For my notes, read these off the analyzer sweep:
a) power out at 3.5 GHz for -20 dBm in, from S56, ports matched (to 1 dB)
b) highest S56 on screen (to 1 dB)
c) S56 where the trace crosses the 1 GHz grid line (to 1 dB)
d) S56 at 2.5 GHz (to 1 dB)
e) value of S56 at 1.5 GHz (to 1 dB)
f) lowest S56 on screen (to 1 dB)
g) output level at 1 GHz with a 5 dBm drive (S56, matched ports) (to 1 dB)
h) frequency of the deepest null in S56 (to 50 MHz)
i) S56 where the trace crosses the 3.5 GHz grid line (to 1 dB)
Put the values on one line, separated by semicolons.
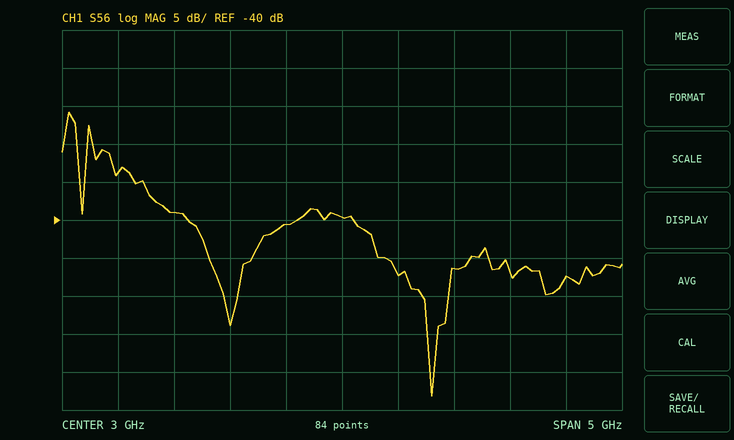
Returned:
-67 dBm; -26 dB; -34 dB; -41 dB; -39 dB; -63 dB; -29 dBm; 3.80 GHz; -47 dB
